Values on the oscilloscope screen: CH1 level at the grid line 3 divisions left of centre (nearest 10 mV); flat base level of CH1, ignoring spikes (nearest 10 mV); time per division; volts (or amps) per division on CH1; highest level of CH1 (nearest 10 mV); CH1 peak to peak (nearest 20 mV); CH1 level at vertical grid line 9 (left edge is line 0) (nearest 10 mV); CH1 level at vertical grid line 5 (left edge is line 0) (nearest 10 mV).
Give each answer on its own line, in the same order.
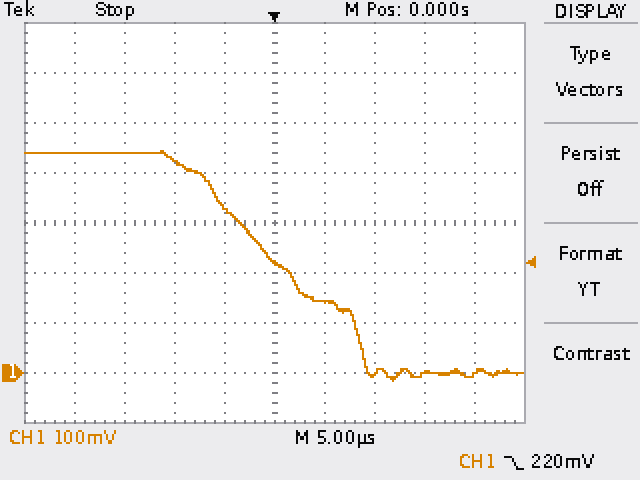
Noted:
440 mV
0 mV
5 µs
100 mV
440 mV
460 mV
0 mV
220 mV
